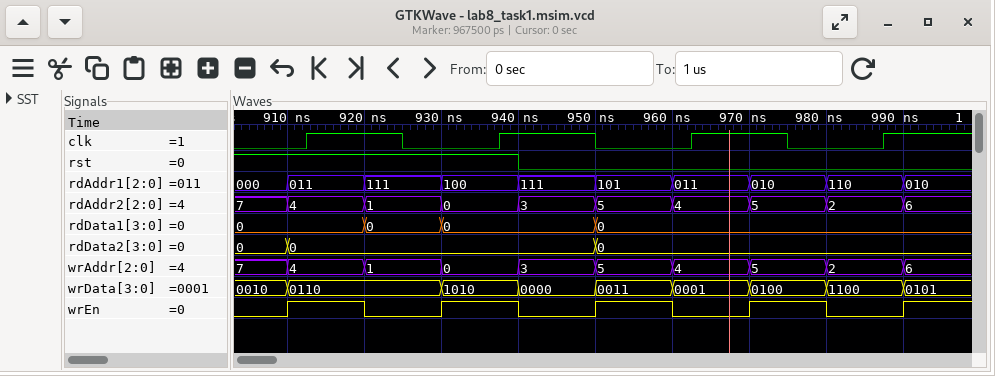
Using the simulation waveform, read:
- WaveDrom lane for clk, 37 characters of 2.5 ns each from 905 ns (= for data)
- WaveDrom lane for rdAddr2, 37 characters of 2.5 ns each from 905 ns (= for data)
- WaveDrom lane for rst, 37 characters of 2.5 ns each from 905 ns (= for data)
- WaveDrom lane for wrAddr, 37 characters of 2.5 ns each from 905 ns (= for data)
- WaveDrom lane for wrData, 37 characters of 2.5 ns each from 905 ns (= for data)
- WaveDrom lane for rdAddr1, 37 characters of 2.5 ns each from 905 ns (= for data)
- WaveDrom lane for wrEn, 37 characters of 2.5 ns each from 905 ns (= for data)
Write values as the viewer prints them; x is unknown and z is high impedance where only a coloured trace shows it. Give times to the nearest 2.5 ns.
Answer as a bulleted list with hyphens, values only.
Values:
- {name: 'clk', wave: '0..1....0....1....0....1....0....1...'}
- {name: 'rdAddr2', wave: '=.=...=...=...=...=...=...=...=...=..', data: '7 4 1 0 3 5 4 5 2 6'}
- {name: 'rst', wave: '1.............0......................'}
- {name: 'wrAddr', wave: '=.=...=...=...=...=...=...=...=...=..', data: '7 4 1 0 3 5 4 5 2 6'}
- {name: 'wrData', wave: '=.=.......=...=...=...=...=...=...=..', data: '0010 0110 1010 0000 0011 0001 0100 1100 0101'}
- {name: 'rdAddr1', wave: '=.=...=...=...=...=...=...=...=...=..', data: '000 011 111 100 111 101 011 010 110 010'}
- {name: 'wrEn', wave: '0.1...0...1...0...1...0...1...0...1..'}
